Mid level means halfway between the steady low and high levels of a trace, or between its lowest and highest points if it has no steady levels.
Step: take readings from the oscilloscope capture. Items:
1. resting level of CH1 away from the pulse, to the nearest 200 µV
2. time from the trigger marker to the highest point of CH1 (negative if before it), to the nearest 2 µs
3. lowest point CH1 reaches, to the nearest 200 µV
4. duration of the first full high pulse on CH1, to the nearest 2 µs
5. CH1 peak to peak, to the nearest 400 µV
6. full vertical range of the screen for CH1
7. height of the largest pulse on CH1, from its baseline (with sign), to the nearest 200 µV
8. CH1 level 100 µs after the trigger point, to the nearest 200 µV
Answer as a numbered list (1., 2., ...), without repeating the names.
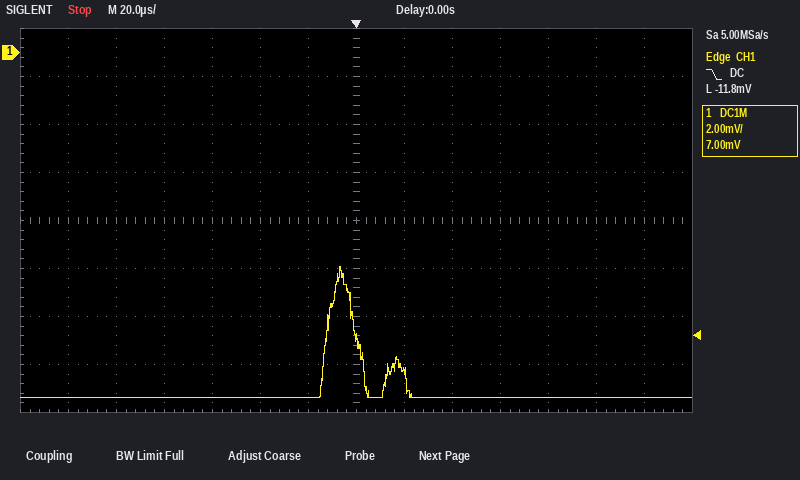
1. -14.4 mV
2. -6 µs
3. -14.4 mV
4. 12 µs
5. 5.6 mV
6. 16 mV
7. +5.4 mV
8. -14.4 mV
